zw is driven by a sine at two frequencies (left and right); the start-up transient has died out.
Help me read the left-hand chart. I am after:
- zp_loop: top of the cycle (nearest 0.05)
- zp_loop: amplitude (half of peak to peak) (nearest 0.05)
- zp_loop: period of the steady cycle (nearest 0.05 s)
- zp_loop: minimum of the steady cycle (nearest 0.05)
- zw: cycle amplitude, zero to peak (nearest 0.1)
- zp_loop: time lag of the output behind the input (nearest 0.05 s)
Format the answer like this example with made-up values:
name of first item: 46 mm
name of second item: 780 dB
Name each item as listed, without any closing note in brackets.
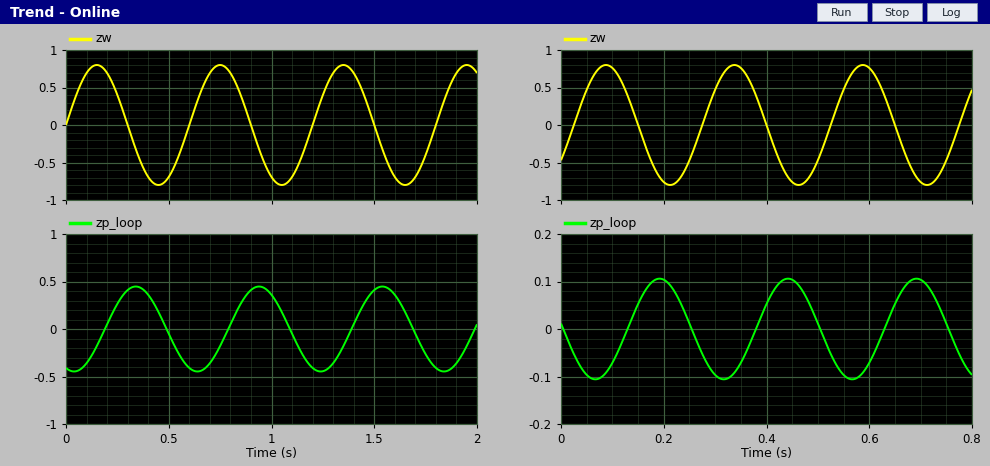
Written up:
zp_loop: top of the cycle: 0.45
zp_loop: amplitude (half of peak to peak): 0.45
zp_loop: period of the steady cycle: 0.60 s
zp_loop: minimum of the steady cycle: -0.45
zw: cycle amplitude, zero to peak: 0.8
zp_loop: time lag of the output behind the input: 0.20 s
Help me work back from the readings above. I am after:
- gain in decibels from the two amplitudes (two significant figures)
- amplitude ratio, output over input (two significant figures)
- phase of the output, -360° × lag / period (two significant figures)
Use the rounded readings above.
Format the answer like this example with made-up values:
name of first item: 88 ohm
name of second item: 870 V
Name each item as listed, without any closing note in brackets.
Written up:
gain in decibels from the two amplitudes: -5.0 dB
amplitude ratio, output over input: 0.56
phase of the output, -360° × lag / period: -120°
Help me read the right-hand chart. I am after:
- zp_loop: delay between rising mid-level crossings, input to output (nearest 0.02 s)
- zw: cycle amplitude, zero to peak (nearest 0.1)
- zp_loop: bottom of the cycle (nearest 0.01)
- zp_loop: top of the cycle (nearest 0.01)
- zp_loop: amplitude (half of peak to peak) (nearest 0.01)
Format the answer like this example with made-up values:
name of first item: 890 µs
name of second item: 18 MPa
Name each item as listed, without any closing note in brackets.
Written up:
zp_loop: delay between rising mid-level crossings, input to output: 0.10 s
zw: cycle amplitude, zero to peak: 0.8
zp_loop: bottom of the cycle: -0.11
zp_loop: top of the cycle: 0.11
zp_loop: amplitude (half of peak to peak): 0.11
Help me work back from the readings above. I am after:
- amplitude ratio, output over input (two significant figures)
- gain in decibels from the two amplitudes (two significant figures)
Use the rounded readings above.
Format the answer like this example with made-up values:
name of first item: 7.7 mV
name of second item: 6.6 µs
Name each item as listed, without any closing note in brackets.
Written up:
amplitude ratio, output over input: 0.14
gain in decibels from the two amplitudes: -17 dB
